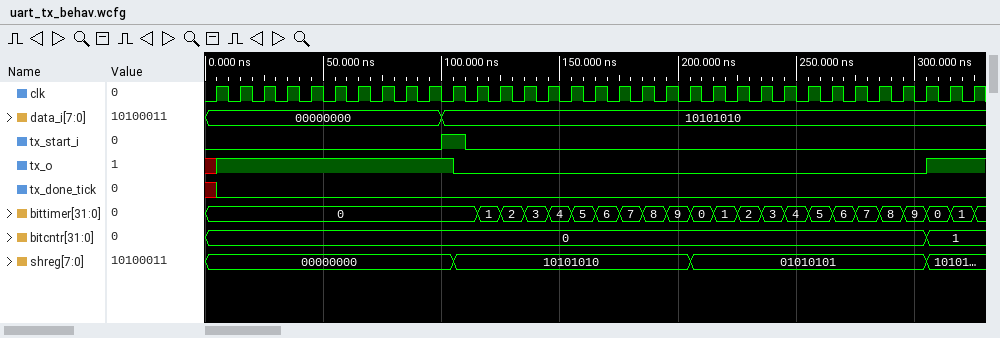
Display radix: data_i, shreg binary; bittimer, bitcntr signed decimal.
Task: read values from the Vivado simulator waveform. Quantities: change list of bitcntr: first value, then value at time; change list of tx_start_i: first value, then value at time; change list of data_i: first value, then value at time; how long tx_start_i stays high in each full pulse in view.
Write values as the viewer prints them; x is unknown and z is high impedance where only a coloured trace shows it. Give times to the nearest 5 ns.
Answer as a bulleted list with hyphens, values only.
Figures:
- 0, 1 at 305 ns
- 0, 1 at 100 ns, 0 at 110 ns
- 00000000, 10101010 at 100 ns
- 10 ns
